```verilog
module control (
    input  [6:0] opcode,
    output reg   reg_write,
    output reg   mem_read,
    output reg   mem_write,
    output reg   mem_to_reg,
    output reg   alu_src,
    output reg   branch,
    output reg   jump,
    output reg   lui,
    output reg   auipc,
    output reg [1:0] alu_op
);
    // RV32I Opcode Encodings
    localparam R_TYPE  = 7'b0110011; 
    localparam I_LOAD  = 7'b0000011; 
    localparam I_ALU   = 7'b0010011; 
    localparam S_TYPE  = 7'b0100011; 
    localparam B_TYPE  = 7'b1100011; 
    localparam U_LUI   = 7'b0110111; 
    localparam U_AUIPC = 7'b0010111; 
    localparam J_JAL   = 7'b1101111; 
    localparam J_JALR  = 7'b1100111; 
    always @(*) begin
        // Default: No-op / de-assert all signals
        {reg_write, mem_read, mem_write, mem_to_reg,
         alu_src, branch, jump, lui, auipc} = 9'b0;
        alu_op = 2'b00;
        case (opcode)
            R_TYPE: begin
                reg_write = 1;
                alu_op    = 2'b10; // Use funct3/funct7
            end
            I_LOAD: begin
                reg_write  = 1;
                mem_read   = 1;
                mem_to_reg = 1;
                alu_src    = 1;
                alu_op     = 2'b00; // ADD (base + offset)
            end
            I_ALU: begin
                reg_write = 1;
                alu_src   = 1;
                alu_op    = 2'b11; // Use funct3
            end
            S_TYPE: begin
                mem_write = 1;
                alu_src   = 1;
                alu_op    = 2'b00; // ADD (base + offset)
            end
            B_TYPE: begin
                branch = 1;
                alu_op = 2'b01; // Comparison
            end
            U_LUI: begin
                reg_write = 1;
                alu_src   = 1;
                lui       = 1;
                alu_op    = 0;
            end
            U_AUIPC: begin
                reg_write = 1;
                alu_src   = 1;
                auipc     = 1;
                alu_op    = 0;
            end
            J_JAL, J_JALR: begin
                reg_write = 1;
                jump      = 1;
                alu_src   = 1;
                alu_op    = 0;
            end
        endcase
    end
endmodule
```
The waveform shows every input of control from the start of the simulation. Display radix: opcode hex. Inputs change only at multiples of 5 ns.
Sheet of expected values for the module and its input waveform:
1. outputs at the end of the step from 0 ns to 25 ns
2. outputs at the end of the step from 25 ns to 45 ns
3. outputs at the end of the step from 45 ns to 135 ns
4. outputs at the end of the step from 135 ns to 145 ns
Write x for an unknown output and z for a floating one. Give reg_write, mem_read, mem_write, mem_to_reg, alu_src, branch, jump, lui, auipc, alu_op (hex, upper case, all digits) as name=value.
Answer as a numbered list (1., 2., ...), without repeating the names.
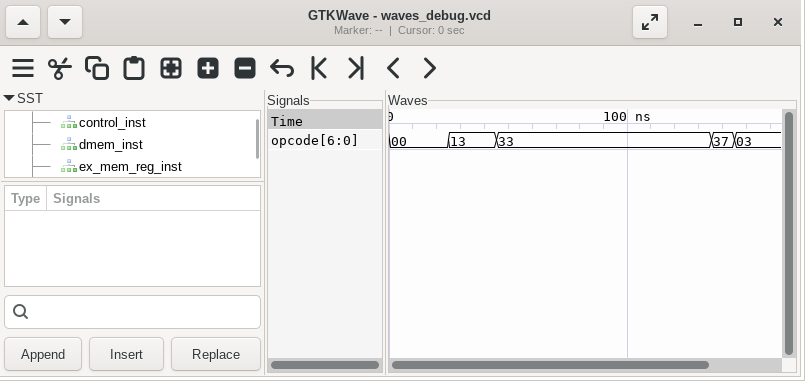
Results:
1. reg_write=0, mem_read=0, mem_write=0, mem_to_reg=0, alu_src=0, branch=0, jump=0, lui=0, auipc=0, alu_op=0
2. reg_write=1, mem_read=0, mem_write=0, mem_to_reg=0, alu_src=1, branch=0, jump=0, lui=0, auipc=0, alu_op=3
3. reg_write=1, mem_read=0, mem_write=0, mem_to_reg=0, alu_src=0, branch=0, jump=0, lui=0, auipc=0, alu_op=2
4. reg_write=1, mem_read=0, mem_write=0, mem_to_reg=0, alu_src=1, branch=0, jump=0, lui=1, auipc=0, alu_op=0
